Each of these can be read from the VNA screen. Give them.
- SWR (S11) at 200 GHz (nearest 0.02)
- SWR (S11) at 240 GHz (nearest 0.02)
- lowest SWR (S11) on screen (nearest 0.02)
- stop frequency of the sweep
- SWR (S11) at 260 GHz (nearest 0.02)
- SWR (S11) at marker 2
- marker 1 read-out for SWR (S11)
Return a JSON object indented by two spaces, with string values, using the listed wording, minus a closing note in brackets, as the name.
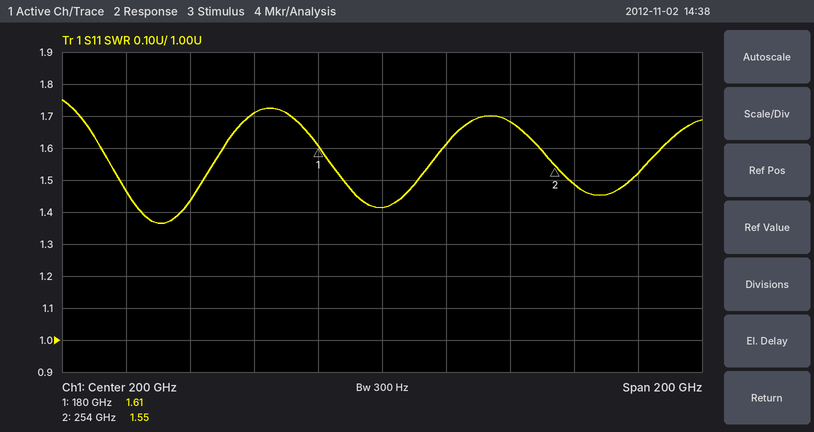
{
  "SWR (S11) at 200 GHz": "1.42",
  "SWR (S11) at 240 GHz": "1.68",
  "lowest SWR (S11) on screen": "1.36",
  "stop frequency of the sweep": "300 GHz",
  "SWR (S11) at 260 GHz": "1.48",
  "SWR (S11) at marker 2": "1.55",
  "marker 1 read-out for SWR": "1.61"
}
